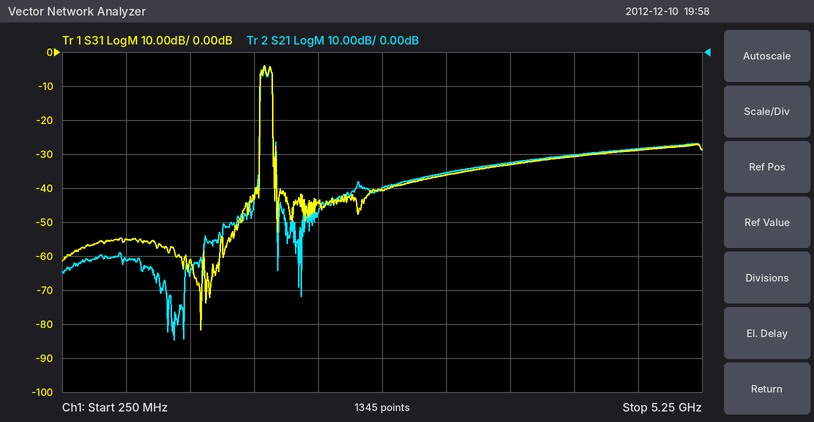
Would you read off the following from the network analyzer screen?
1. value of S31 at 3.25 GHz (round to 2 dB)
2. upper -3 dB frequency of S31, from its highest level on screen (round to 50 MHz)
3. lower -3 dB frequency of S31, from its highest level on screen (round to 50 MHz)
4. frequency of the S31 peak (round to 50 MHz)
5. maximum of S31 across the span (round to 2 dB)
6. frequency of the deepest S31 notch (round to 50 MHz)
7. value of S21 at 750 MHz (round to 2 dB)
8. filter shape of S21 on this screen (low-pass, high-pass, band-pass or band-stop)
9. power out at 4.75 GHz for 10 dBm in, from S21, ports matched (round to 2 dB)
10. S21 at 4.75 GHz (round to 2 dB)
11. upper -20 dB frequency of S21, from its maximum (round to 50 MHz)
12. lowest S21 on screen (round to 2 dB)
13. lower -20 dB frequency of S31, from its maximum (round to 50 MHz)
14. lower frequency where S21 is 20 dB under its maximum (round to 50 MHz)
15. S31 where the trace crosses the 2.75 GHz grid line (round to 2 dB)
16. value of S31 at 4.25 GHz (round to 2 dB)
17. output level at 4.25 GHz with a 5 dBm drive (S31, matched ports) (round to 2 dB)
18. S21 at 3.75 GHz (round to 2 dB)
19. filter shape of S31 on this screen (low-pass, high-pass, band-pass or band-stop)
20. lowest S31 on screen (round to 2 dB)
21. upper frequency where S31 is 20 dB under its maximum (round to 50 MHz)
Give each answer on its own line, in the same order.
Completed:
-36 dB
1.90 GHz
1.80 GHz
1.85 GHz
-4 dB
1.35 GHz
-62 dB
band-pass
-18 dBm
-28 dB
1.90 GHz
-84 dB
1.80 GHz
1.80 GHz
-40 dB
-30 dB
-26 dBm
-32 dB
band-pass
-82 dB
1.90 GHz
